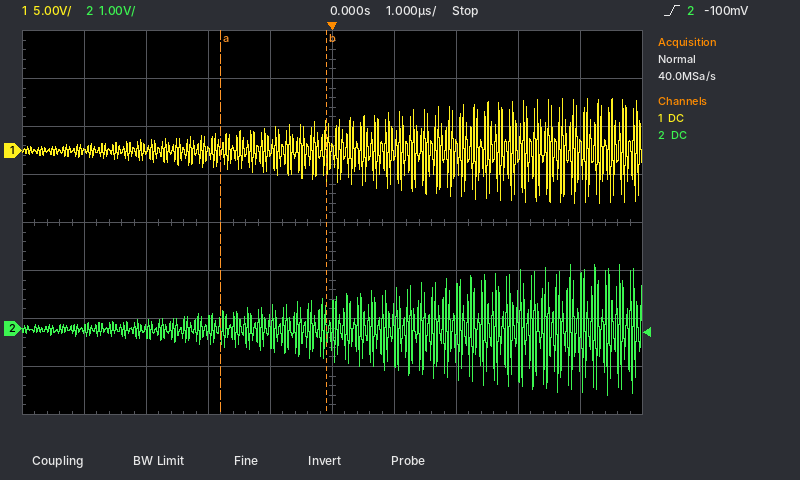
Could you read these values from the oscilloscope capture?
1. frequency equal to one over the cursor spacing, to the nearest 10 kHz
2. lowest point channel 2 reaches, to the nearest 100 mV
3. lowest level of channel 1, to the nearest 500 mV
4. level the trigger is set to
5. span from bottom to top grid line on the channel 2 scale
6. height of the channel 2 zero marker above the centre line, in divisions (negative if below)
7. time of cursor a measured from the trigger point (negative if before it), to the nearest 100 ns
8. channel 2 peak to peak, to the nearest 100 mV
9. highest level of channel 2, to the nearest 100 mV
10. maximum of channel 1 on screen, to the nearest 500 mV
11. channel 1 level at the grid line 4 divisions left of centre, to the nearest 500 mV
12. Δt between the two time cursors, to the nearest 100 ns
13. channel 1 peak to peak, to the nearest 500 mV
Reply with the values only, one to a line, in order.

590 kHz
-1.4 V
-5.5 V
-100 mV
8 V
-2.2 div
-1.8 µs
2.7 V
1.3 V
5.5 V
0.0 V
1.7 µs
11.0 V
